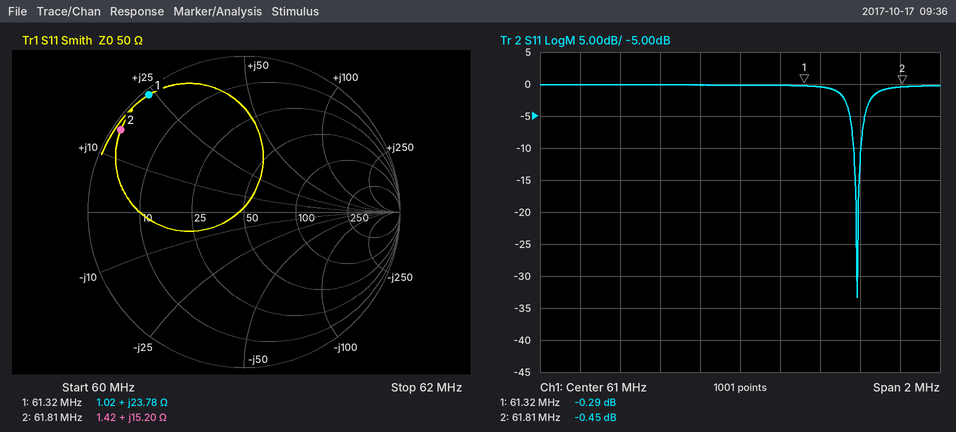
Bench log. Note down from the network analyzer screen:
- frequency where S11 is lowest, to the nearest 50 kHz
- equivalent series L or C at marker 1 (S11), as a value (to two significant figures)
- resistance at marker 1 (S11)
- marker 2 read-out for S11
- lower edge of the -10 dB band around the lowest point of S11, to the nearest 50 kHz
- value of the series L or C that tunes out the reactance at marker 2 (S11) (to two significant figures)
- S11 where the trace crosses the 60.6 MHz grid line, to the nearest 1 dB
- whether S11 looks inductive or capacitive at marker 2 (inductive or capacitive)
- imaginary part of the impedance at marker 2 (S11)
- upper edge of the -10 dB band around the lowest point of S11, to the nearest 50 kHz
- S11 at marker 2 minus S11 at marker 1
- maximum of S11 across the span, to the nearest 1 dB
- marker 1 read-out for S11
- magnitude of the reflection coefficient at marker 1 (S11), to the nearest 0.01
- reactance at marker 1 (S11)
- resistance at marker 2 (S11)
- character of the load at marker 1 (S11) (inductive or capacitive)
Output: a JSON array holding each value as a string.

["61.60 MHz", "62 nH", "1.02 Ω", "-0.45 dB", "61.55 MHz", "170 pF", "0 dB", "inductive", "+15.20 Ω", "61.60 MHz", "-0.16 dB", "0 dB", "-0.29 dB", "0.97", "+23.78 Ω", "1.42 Ω", "inductive"]
